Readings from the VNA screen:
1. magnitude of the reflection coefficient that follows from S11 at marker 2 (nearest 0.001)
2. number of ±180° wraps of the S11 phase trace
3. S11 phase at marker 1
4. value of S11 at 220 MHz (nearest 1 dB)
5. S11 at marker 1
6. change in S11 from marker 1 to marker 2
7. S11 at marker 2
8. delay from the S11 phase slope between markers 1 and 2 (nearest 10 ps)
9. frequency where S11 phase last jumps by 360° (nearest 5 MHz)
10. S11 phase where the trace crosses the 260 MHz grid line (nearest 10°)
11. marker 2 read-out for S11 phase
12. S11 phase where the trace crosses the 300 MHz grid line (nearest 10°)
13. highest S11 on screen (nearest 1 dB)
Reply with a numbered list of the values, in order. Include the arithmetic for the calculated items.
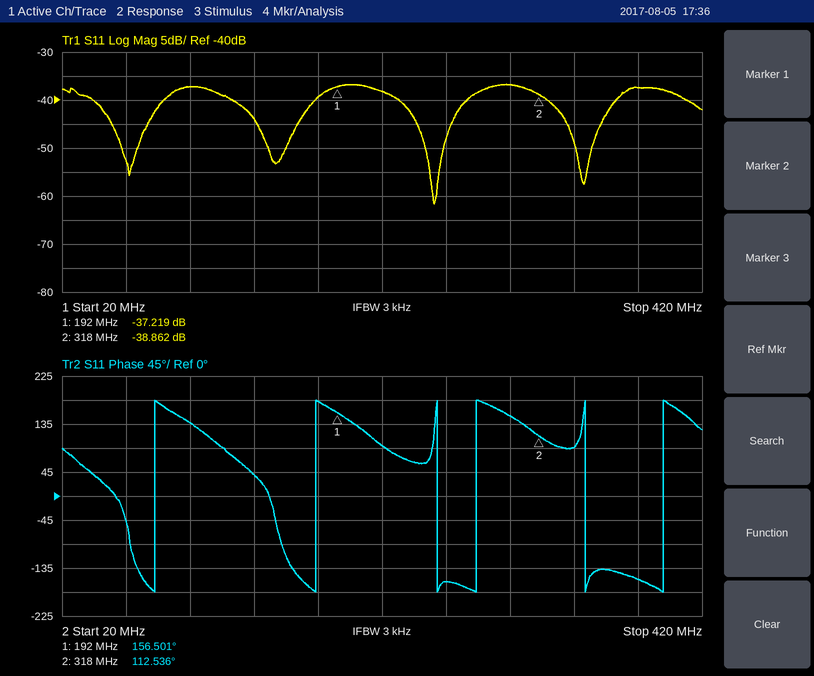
1. 10^(-38.862/20) ≈ 0.011
2. 6
3. 156.501°
4. -38 dB
5. -37.219 dB
6. -38.862 − (-37.219) = -1.643 dB
7. -38.862 dB
8. −(112.536° − (156.501°))/(360° × 126 MHz) ≈ 969 ps, so 970 ps to the nearest 10 ps
9. 395 MHz
10. -160°
11. 112.536°
12. 150°
13. -37 dB
